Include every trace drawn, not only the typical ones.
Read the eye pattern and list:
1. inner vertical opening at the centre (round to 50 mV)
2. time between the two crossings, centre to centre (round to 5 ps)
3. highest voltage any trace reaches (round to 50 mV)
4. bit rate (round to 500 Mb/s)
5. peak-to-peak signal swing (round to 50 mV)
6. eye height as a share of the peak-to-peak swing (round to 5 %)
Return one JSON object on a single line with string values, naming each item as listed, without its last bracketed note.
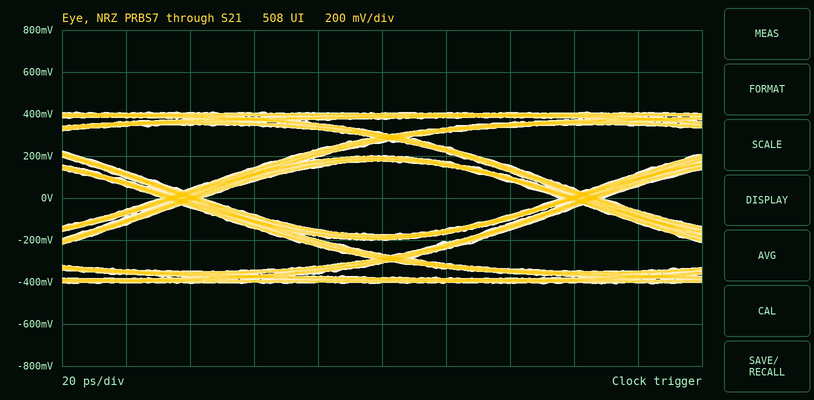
{"inner vertical opening at the centre": "350 mV", "time between the two crossings, centre to centre": "125 ps", "highest voltage any trace reaches": "400 mV", "bit rate": "8.0 Gb/s", "peak-to-peak signal swing": "800 mV", "eye height as a share of the peak-to-peak swing": "45 %"}
